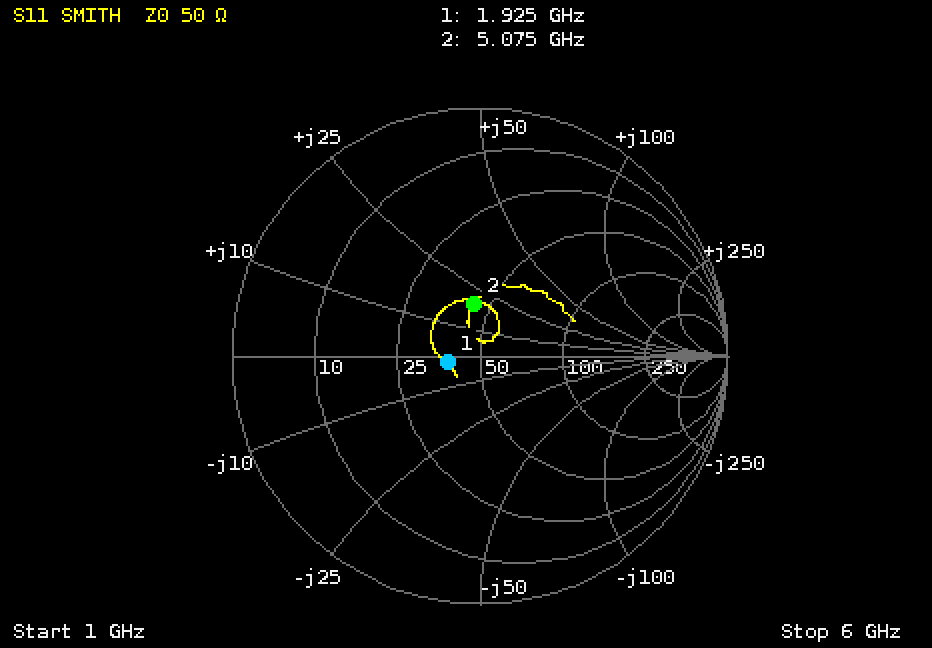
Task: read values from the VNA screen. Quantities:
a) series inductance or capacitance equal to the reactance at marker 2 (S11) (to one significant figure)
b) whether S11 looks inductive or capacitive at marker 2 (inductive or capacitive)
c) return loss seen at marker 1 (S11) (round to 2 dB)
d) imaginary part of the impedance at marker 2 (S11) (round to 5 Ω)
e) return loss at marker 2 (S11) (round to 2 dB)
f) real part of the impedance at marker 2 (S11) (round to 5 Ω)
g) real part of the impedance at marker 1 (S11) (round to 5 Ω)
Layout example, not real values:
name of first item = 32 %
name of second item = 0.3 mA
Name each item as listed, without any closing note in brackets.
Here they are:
series inductance or capacitance equal to the reactance at marker 2 (S11) = 600 pH
whether S11 looks inductive or capacitive at marker 2 = inductive
return loss seen at marker 1 (S11) = 18 dB
imaginary part of the impedance at marker 2 (S11) = +20 Ω
return loss at marker 2 (S11) = 14 dB
real part of the impedance at marker 2 (S11) = 45 Ω
real part of the impedance at marker 1 (S11) = 40 Ω
